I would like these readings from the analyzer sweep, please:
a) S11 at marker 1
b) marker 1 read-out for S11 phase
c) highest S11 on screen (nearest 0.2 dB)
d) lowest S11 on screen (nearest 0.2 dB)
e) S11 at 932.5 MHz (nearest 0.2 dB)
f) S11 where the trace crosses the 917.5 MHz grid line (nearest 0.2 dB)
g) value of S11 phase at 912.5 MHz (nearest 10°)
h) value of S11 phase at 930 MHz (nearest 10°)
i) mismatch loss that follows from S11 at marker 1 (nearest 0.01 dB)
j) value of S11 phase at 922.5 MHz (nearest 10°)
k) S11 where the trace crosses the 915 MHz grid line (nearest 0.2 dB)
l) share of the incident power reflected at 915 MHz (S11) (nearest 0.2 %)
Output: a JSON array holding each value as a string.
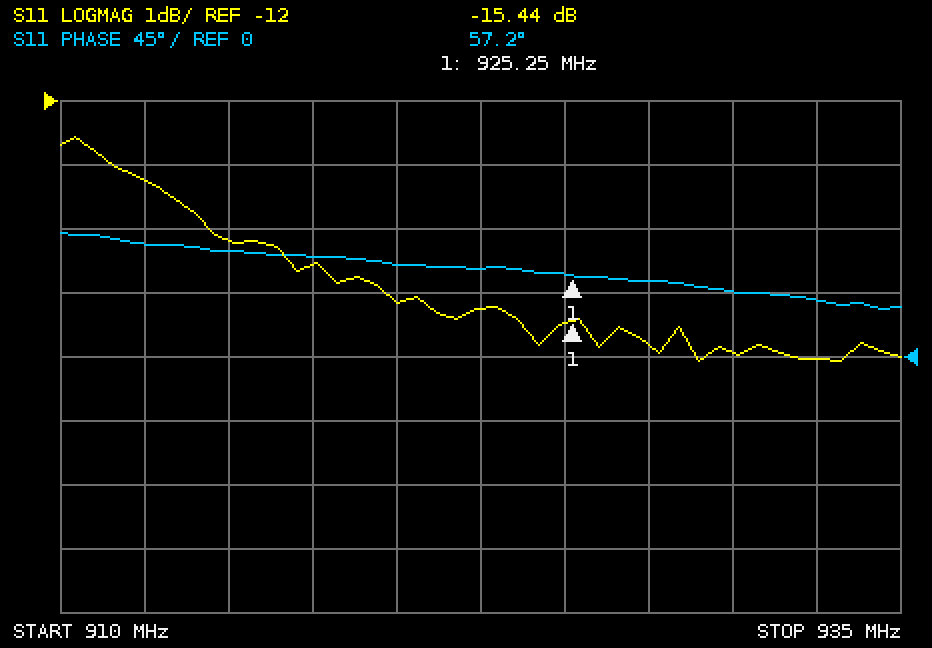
["-15.44 dB", "57.2°", "-12.6 dB", "-16.0 dB", "-16.0 dB", "-14.6 dB", "80°", "50°", "0.13 dB", "60°", "-14.2 dB", "3.8 %"]
